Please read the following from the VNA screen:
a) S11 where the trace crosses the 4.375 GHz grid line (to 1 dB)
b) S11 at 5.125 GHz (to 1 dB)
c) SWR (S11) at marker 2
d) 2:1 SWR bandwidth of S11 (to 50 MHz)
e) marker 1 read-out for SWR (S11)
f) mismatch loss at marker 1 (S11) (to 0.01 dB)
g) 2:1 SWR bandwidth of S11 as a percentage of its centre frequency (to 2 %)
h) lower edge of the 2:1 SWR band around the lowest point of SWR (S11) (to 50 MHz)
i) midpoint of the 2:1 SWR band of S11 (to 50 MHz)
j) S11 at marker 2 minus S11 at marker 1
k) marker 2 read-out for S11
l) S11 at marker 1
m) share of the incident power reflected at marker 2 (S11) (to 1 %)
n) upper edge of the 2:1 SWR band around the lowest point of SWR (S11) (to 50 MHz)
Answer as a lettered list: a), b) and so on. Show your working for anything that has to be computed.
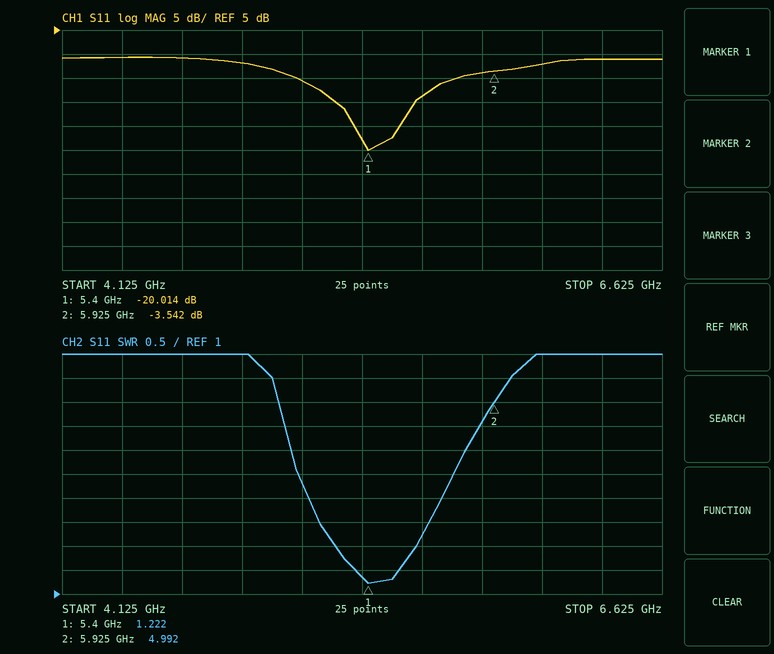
a) -1 dB
b) -6 dB
c) 4.992
d) 5.60 GHz − 5.25 GHz = 350 MHz
e) 1.222
f) −10 log10(1 − 10^(-20.014/10)) ≈ 0.04 dB
g) 350 MHz / 5.425 GHz ≈ 6 %
h) 5.25 GHz
i) 5.45 GHz
j) -3.542 − (-20.014) = 16.472 dB
k) -3.542 dB
l) -20.014 dB
m) 10^(-3.542/10) ≈ 44 %
n) 5.60 GHz
